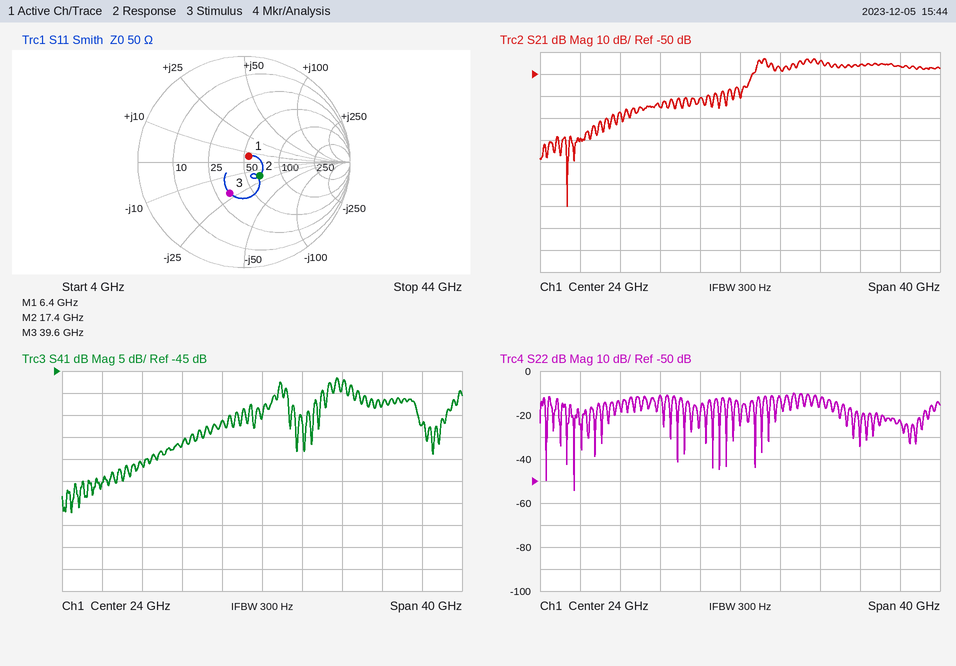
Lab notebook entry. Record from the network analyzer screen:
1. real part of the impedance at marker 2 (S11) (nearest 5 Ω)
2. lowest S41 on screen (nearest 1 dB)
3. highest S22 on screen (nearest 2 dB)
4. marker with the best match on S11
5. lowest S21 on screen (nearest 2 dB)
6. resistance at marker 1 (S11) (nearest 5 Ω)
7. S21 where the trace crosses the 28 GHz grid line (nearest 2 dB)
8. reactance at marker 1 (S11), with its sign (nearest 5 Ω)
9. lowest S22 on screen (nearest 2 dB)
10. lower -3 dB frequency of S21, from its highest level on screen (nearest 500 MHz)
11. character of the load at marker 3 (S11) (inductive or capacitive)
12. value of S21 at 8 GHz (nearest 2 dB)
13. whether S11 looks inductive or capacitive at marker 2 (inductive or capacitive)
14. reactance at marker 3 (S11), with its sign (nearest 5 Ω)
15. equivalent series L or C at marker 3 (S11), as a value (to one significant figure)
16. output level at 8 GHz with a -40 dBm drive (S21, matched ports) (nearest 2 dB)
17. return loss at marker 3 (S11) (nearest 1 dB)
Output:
65 Ω
-77 dB
-10 dB
marker 1
-110 dB
55 Ω
-48 dB
+5 Ω
-54 dB
25.5 GHz
capacitive
-80 dB
capacitive
-20 Ω
200 fF
-120 dBm
10 dB
